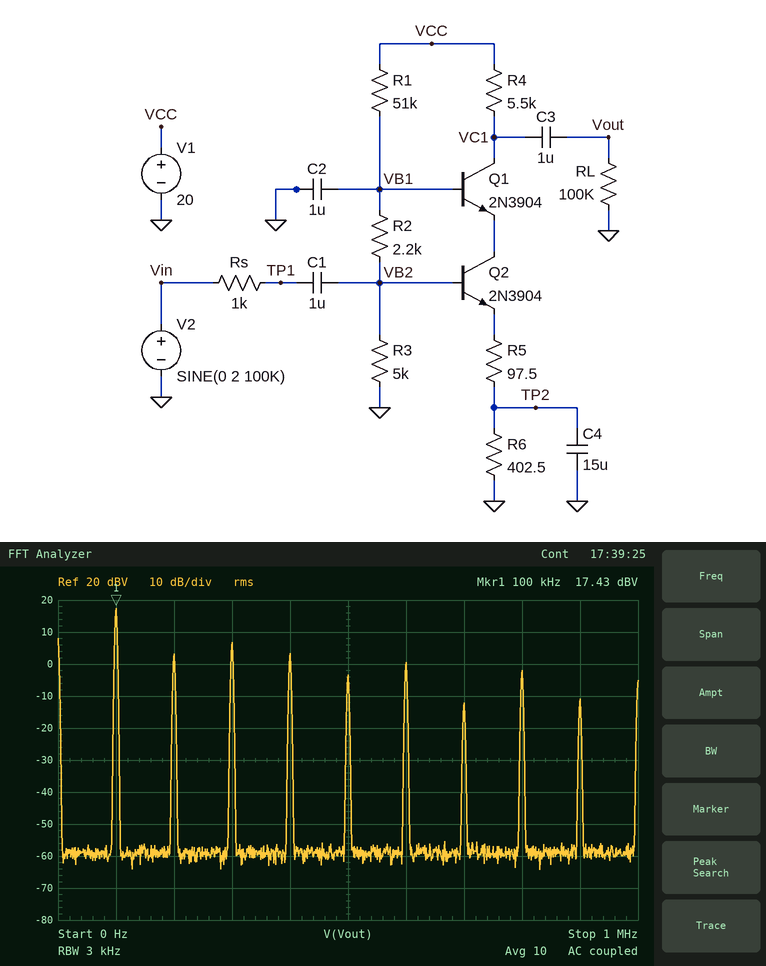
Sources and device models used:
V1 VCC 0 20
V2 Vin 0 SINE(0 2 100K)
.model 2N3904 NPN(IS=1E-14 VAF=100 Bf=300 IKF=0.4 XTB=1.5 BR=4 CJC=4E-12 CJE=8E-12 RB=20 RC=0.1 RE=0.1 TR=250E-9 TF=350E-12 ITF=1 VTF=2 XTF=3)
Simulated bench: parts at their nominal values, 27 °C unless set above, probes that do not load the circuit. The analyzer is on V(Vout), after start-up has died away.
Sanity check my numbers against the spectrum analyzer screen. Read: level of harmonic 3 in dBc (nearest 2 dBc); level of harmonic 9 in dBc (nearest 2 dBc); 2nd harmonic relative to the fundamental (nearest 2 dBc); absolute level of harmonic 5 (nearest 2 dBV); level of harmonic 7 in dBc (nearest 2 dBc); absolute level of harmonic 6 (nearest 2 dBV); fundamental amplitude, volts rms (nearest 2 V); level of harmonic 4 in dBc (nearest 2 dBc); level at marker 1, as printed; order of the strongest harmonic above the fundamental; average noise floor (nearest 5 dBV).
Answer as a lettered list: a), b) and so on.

a) -10 dBc
b) -28 dBc
c) -14 dBc
d) -4 dBV
e) -30 dBc
f) 0 dBV
g) 8 V
h) -14 dBc
i) 17.43 dBV
j) 3
k) -60 dBV
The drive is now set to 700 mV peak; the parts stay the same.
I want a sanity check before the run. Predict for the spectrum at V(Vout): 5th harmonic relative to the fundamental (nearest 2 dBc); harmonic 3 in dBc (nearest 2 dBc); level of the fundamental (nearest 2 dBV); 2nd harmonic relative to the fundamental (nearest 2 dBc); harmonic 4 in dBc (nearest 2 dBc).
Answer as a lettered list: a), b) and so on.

a) -30 dBc
b) -16 dBc
c) 18 dBV
d) -12 dBc
e) -18 dBc
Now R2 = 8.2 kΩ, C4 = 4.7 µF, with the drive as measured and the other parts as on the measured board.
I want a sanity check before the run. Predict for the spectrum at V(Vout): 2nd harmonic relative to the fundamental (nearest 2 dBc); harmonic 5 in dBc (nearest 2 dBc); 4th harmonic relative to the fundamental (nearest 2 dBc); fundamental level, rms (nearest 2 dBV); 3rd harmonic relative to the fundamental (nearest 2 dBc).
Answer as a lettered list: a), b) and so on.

a) -8 dBc
b) -18 dBc
c) -12 dBc
d) 18 dBV
e) -20 dBc
